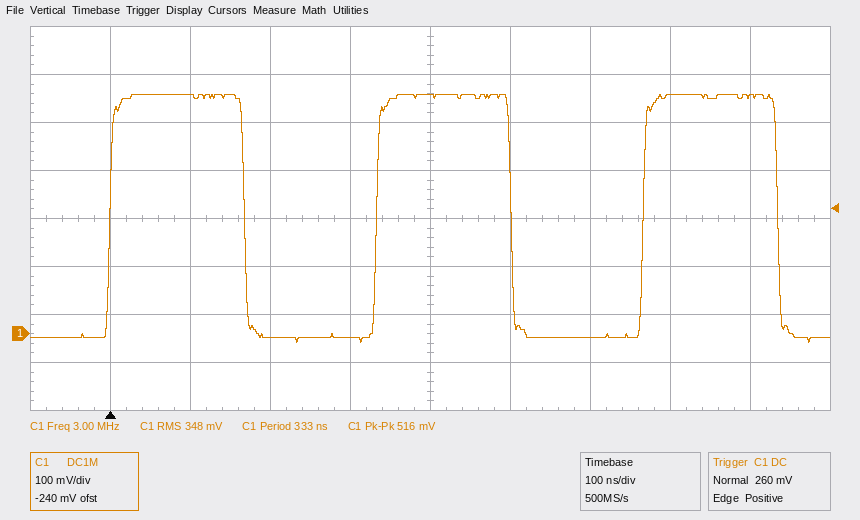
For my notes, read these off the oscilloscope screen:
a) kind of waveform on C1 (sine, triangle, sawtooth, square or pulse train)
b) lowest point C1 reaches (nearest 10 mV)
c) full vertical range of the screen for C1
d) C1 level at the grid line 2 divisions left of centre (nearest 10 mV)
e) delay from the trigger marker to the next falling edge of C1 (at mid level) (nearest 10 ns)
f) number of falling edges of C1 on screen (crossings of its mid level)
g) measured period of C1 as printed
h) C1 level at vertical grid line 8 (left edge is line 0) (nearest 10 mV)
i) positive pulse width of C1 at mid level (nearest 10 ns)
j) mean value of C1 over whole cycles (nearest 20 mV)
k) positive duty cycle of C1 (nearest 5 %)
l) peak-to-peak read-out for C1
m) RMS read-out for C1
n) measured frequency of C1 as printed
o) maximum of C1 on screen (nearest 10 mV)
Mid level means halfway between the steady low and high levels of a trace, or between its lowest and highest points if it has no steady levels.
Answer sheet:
square
-20 mV
800 mV
-10 mV
170 ns
3
333 ns
500 mV
170 ns
240 mV
50 %
516 mV
348 mV
3.00 MHz
500 mV
